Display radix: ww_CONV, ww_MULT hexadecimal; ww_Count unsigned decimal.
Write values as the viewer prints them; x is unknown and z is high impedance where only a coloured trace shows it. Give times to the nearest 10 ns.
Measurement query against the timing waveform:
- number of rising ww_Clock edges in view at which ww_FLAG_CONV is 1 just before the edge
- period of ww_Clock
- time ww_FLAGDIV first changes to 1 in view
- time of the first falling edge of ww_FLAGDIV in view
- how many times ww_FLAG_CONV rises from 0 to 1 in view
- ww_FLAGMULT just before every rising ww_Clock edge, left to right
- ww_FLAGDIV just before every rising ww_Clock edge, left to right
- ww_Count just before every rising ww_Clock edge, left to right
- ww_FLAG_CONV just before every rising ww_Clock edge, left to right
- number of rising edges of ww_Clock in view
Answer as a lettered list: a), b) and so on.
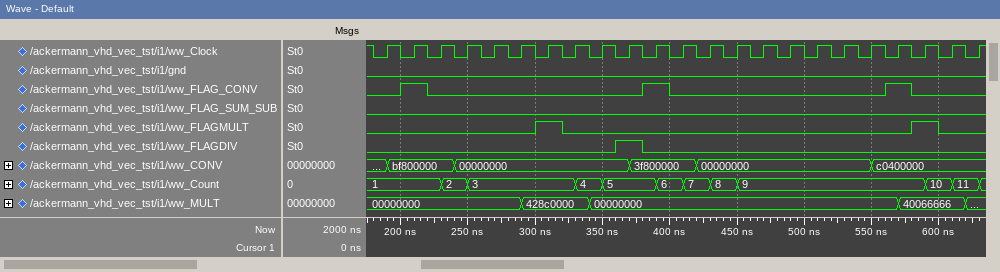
a) 3
b) 20 ns
c) 360 ns
d) 380 ns
e) 3
f) 0 0 0 0 0 0 1 0 0 0 0 0 0 0 0 0 0 0 0 0 1 0 0
g) 0 0 0 0 0 0 0 0 0 1 0 0 0 0 0 0 0 0 0 0 0 0 0
h) 1, 1, 1, 2, 3, 3, 3, 3, 4, 5, 5, 6, 7, 8, 9, 9, 9, 9, 9, 9, 9, 10, 11
i) 0 1 0 0 0 0 0 0 0 0 1 0 0 0 0 0 0 0 0 1 0 0 0
j) 23
